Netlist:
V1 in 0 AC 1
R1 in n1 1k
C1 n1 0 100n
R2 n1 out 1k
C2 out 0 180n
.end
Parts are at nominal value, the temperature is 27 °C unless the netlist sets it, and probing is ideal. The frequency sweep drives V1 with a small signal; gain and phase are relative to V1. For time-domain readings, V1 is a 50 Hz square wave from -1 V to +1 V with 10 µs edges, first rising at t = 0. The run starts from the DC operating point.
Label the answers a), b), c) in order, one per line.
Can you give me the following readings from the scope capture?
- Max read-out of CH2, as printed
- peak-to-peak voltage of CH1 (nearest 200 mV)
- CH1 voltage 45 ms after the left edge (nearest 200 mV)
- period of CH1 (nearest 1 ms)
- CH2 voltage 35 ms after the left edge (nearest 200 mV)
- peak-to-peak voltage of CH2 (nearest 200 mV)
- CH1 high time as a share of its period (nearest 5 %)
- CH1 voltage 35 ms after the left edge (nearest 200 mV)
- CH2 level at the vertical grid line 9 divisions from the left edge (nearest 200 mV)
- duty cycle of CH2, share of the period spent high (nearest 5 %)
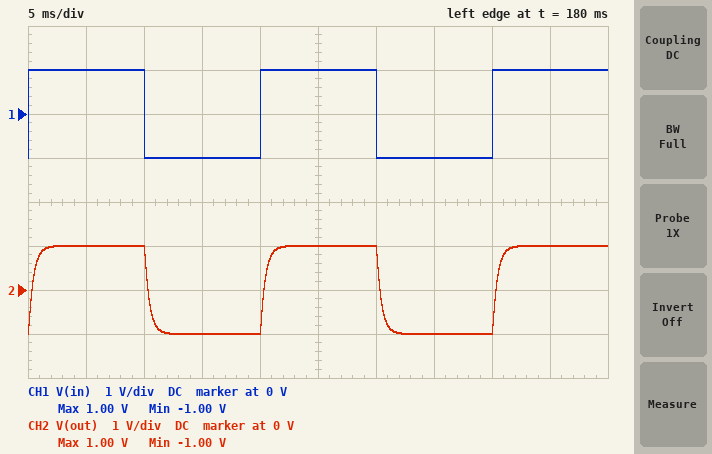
a) 1.00 V
b) 2.0 V
c) 1.0 V
d) 20 ms
e) -1.0 V
f) 2.0 V
g) 50 %
h) -1.0 V
i) 1.0 V
j) 50 %
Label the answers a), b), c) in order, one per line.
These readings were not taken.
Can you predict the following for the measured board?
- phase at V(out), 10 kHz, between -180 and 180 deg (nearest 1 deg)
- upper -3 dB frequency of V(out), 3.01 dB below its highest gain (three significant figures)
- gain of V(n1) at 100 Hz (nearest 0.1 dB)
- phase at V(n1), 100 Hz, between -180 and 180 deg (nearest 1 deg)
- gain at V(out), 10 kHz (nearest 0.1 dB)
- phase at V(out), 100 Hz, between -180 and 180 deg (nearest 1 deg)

a) -158 deg
b) 378 Hz
c) -0.2 dB
d) -10 deg
e) -37.6 dB
f) -16 deg
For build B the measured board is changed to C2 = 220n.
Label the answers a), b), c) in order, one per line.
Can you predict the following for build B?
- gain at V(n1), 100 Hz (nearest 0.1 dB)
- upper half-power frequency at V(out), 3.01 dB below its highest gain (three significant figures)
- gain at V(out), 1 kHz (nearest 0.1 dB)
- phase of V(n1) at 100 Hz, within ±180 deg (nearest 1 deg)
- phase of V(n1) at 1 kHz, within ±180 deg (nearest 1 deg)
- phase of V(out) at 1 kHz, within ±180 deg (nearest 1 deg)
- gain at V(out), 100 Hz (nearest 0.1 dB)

a) -0.3 dB
b) 319 Hz
c) -10.6 dB
d) -11 deg
e) -34 deg
f) -88 deg
g) -0.4 dB
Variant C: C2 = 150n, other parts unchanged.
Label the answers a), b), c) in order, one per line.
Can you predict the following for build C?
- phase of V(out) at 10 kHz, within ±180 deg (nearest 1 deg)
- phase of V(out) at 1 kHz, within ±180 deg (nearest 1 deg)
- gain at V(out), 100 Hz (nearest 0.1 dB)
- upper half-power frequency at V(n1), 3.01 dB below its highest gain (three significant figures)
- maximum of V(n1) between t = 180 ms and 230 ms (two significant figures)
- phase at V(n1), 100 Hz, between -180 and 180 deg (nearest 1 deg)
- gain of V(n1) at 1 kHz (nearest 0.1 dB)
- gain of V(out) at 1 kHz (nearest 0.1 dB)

a) -157 deg
b) -81 deg
c) -0.2 dB
d) 538 Hz
e) 1.0 V
f) -9 deg
g) -5.4 dB
h) -8.1 dB
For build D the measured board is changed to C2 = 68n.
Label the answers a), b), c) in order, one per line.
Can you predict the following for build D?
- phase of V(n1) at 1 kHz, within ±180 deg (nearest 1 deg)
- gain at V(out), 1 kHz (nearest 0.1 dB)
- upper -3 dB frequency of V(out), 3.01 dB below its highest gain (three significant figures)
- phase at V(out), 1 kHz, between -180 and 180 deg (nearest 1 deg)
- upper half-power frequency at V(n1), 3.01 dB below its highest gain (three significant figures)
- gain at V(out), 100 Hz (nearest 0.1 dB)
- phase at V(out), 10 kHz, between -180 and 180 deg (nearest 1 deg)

a) -41 deg
b) -4.4 dB
c) 766 Hz
d) -64 deg
e) 861 Hz
f) -0.1 dB
g) -150 deg
